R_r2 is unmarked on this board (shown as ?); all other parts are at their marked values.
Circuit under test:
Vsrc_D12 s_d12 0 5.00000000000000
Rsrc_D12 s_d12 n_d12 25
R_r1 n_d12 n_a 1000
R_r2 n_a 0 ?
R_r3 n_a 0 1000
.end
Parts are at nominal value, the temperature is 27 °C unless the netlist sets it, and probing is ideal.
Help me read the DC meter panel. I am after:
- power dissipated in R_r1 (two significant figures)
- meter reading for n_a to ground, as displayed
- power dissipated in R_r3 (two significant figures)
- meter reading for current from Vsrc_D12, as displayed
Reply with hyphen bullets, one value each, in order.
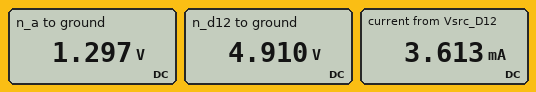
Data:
- 13 mW
- 1.297 V
- 1.7 mW
- 3.613 mA
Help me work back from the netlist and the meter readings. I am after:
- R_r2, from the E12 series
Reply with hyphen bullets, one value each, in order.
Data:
- 560 Ω
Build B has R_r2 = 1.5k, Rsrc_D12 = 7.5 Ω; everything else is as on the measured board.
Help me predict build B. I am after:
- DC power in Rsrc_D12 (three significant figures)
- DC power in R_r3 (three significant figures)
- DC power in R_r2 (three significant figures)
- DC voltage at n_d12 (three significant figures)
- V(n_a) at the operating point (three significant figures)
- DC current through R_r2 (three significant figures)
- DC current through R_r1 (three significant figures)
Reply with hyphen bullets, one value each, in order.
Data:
- 72.6 µW
- 3.48 mW
- 2.32 mW
- 4.98 V
- 1.87 V
- 1.24 mA
- 3.11 mA
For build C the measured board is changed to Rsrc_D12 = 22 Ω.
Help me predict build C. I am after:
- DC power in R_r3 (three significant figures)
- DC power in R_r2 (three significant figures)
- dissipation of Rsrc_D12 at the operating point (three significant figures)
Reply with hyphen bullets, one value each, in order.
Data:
- 1.69 mW
- 3.02 mW
- 288 µW
